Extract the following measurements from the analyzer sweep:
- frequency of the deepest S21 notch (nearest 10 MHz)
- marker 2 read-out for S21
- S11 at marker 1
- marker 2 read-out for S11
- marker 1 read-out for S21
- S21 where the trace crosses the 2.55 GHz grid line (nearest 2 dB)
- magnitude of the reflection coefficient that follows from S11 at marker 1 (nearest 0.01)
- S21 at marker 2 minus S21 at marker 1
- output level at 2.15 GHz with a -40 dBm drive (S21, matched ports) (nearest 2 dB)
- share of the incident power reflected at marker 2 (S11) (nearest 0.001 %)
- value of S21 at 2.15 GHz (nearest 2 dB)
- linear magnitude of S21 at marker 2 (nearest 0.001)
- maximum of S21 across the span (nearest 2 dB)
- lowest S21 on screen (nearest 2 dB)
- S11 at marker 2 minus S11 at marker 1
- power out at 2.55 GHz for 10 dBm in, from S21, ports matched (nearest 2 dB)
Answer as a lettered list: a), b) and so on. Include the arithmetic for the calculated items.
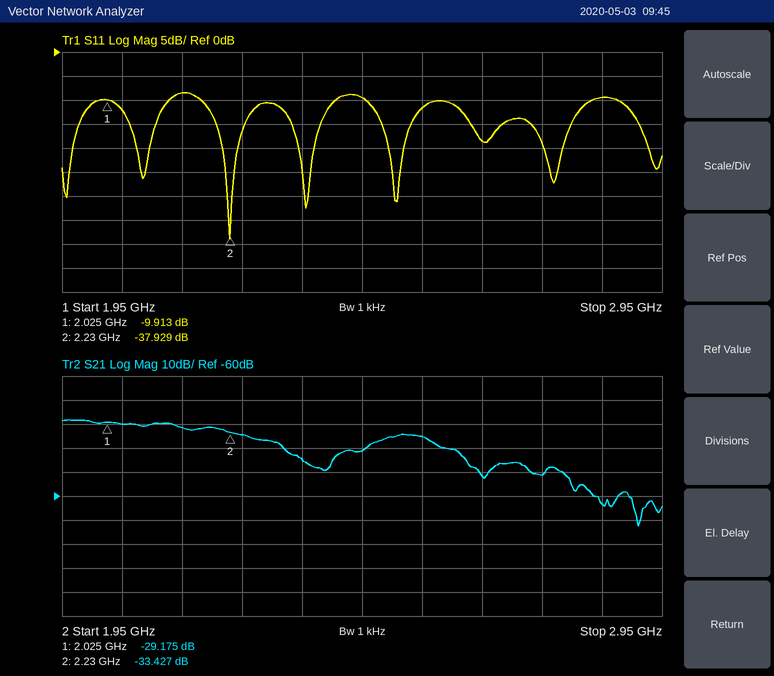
a) 2.91 GHz
b) -33.427 dB
c) -9.913 dB
d) -37.929 dB
e) -29.175 dB
f) -36 dB
g) 10^(-9.913/20) ≈ 0.32
h) -33.427 − (-29.175) = -4.252 dB
i) -40 dBm + (-32 dB) = -72 dBm
j) 10^(-37.929/10) ≈ 0.016 %
k) -32 dB
l) 10^(-33.427/20) ≈ 0.021
m) -28 dB
n) -72 dB
o) -37.929 − (-9.913) = -28.016 dB
p) 10 dBm + (-36 dB) = -26 dBm
